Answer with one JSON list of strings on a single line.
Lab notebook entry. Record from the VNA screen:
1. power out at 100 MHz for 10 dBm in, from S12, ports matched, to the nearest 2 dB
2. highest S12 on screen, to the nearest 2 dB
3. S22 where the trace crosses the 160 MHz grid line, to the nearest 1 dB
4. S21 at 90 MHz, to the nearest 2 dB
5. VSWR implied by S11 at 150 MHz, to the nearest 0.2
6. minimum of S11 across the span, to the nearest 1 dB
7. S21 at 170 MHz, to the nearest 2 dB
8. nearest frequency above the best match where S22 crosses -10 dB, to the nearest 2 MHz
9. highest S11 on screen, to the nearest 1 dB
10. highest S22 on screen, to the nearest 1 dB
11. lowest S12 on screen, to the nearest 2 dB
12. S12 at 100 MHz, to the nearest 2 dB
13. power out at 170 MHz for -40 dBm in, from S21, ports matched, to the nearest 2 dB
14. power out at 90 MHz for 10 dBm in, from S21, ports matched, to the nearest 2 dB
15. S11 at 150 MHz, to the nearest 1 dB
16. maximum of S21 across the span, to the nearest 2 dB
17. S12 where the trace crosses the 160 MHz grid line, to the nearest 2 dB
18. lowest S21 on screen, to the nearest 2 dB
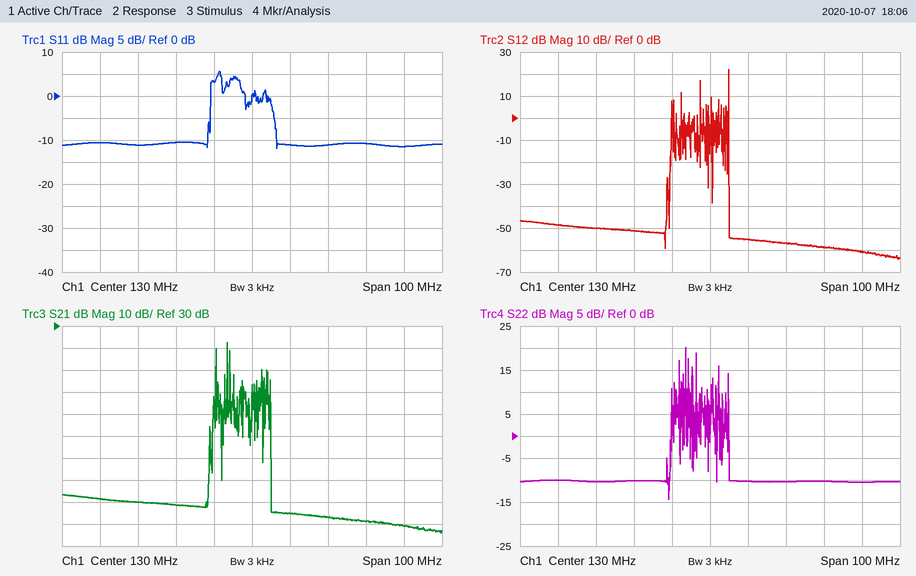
["-40 dBm", "22 dB", "-10 dB", "-48 dB", "1.8", "-12 dB", "-60 dB", "120 MHz", "6 dB", "20 dB", "-64 dB", "-50 dB", "-100 dBm", "-38 dBm", "-11 dB", "22 dB", "-58 dB", "-64 dB"]
